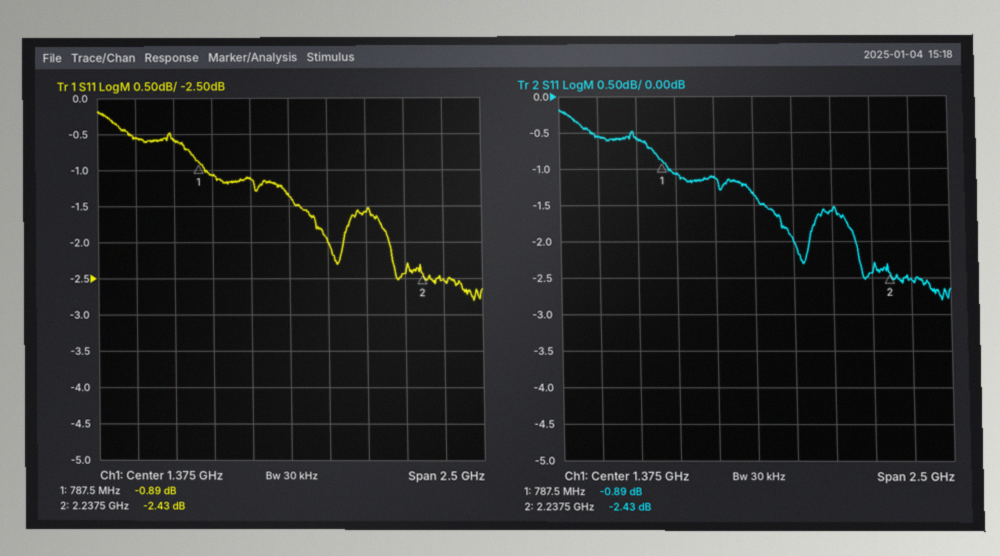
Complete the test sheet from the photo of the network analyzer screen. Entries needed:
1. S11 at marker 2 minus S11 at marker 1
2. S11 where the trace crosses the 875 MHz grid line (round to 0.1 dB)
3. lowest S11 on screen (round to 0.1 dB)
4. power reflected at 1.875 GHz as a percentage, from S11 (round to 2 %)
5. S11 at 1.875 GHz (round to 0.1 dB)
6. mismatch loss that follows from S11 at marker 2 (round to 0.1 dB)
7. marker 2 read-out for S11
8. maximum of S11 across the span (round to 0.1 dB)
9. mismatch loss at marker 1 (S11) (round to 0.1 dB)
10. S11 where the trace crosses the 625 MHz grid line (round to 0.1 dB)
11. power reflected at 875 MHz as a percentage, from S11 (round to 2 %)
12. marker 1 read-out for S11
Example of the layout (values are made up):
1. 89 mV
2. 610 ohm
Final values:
1. -1.54 dB
2. -1.1 dB
3. -2.8 dB
4. 70 %
5. -1.6 dB
6. 3.7 dB
7. -2.43 dB
8. -0.2 dB
9. 7.3 dB
10. -0.6 dB
11. 78 %
12. -0.89 dB
